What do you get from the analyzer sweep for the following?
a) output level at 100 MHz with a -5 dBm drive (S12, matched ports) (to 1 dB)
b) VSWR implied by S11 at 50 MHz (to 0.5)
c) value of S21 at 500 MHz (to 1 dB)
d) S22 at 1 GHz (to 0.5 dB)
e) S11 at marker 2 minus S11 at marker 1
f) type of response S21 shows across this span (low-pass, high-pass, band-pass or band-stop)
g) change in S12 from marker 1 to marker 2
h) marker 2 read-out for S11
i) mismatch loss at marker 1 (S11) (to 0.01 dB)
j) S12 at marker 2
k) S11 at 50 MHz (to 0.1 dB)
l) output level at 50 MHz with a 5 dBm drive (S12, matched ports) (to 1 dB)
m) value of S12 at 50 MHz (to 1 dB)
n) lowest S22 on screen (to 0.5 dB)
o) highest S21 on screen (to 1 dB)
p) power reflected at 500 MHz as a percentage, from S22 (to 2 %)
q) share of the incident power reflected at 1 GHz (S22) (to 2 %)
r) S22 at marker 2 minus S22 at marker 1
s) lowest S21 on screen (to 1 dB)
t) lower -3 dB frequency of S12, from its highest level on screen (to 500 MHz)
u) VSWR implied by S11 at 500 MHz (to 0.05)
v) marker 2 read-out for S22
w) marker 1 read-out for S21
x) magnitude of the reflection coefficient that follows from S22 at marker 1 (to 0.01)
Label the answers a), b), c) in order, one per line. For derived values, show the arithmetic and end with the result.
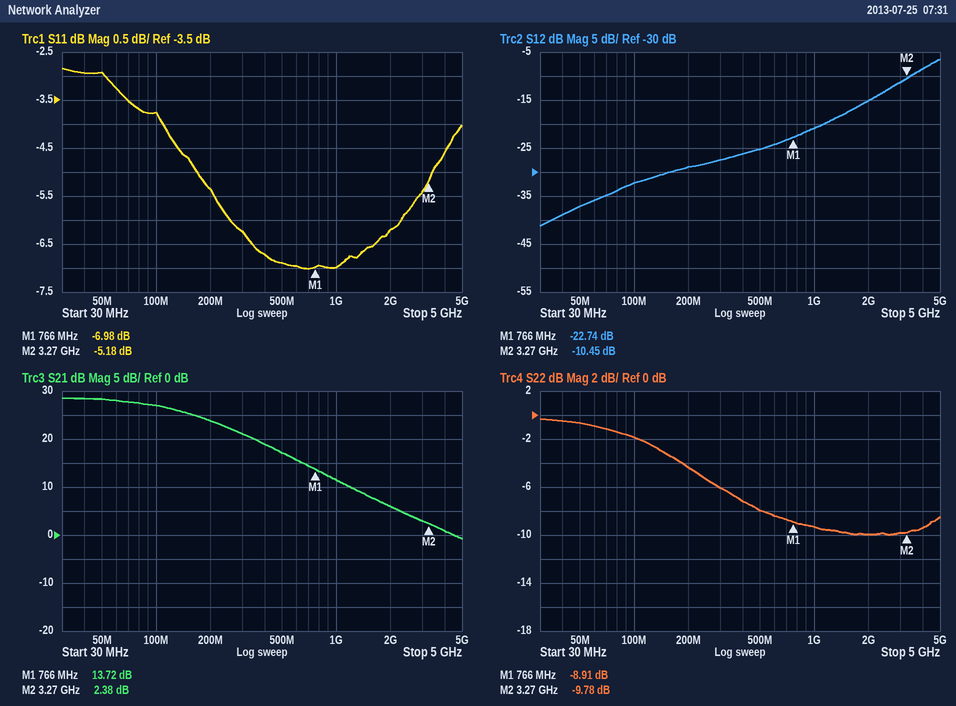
a) -5 dBm + (-32 dB) = -37 dBm
b) |Γ| = 10^(-2.9/20) = 0.7161; VSWR = (1 + 0.7161)/(1 − 0.7161) ≈ 6.0
c) 17 dB
d) -9.5 dB
e) -5.18 − (-6.98) = 1.80 dB
f) low-pass
g) -10.45 − (-22.74) = 12.29 dB
h) -5.18 dB
i) −10 log10(1 − 10^(-6.98/10)) ≈ 0.97 dB
j) -10.45 dB
k) -2.9 dB
l) 5 dBm + (-37 dB) = -32 dBm
m) -37 dB
n) -10.0 dB
o) 29 dB
p) 10^(-8/10) ≈ 16 %
q) 10^(-9.5/10) ≈ 11.2 %, so 12 % to the nearest 2 %
r) -9.78 − (-8.91) = -0.87 dB
s) -1 dB
t) 3.5 GHz
u) |Γ| = 10^(-6.9/20) = 0.4519; VSWR = (1 + 0.4519)/(1 − 0.4519) ≈ 2.65
v) -9.78 dB
w) 13.72 dB
x) 10^(-8.91/20) ≈ 0.36
